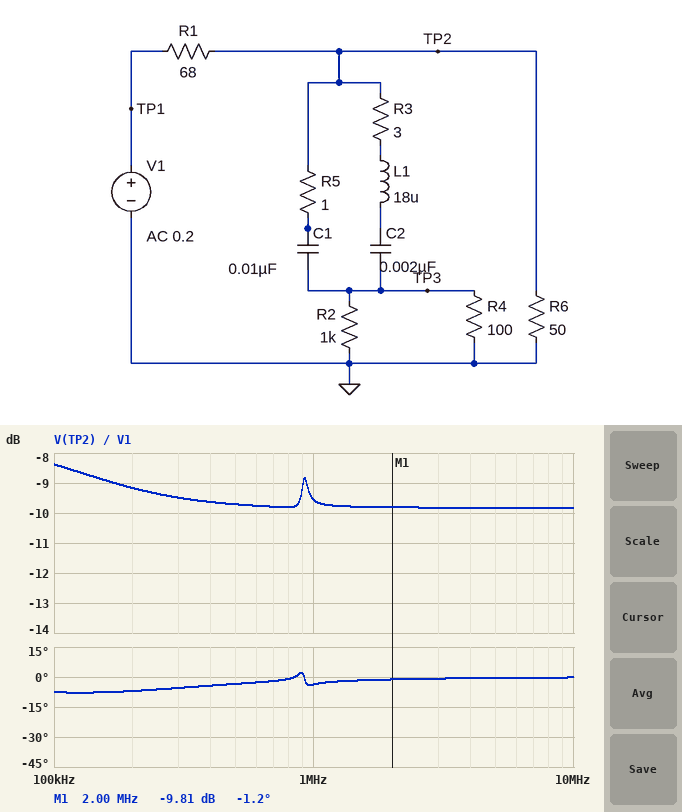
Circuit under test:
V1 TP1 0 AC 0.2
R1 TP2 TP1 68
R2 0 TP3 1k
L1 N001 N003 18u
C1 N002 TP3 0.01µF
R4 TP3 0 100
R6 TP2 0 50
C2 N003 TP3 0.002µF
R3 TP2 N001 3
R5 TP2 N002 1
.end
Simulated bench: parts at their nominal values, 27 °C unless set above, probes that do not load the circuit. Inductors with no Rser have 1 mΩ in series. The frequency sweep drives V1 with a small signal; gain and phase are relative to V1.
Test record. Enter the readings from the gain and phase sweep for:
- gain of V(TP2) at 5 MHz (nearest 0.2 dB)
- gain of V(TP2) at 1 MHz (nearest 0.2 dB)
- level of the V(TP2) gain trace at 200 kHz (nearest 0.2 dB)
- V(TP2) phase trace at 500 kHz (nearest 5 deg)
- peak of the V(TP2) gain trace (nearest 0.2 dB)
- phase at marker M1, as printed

-9.8 dB
-9.6 dB
-9.2 dB
-5 deg
-8.4 dB
-1.2 deg
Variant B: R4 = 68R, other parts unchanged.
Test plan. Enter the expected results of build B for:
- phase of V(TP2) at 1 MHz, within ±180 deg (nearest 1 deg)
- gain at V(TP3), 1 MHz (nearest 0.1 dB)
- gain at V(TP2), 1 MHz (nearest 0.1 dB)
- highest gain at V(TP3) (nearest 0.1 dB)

-6 deg
-11.6 dB
-10.1 dB
-10.8 dB
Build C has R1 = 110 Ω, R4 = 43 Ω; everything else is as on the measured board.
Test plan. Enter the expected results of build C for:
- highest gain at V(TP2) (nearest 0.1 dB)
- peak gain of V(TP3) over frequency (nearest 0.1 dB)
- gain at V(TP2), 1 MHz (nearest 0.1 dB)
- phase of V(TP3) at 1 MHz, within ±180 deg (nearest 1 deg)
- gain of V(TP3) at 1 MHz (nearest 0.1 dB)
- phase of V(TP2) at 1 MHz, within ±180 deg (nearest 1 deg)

-10.1 dB
-15.5 dB
-14.0 dB
20 deg
-16.5 dB
-12 deg
